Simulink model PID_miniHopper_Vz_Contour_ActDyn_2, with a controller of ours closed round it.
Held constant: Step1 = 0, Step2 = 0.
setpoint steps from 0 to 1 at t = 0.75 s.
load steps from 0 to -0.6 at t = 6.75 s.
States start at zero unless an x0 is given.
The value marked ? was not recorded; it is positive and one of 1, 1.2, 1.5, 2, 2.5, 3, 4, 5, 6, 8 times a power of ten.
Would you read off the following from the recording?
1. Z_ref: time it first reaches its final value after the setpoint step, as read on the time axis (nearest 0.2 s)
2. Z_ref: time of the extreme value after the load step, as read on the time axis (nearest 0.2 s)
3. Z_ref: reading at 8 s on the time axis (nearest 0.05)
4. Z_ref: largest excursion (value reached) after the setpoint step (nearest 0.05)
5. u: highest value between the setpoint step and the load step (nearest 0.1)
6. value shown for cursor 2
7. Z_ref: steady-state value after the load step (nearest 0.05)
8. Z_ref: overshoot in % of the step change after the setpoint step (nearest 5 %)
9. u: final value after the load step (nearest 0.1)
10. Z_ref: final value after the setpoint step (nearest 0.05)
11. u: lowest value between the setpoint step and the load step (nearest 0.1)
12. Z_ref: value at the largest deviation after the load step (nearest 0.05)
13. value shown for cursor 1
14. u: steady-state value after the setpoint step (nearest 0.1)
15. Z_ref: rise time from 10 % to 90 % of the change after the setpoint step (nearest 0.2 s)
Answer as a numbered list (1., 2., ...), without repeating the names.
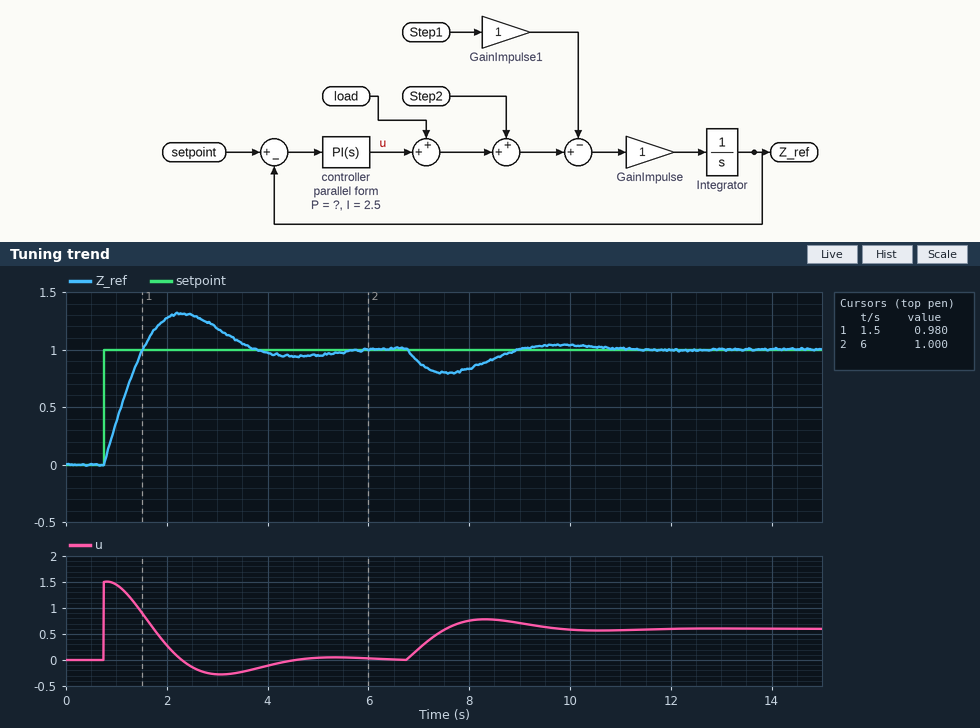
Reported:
1. 1.6 s
2. 7.6 s
3. 0.85
4. 1.30
5. 1.5
6. 1.000
7. 1.00
8. 30 %
9. 0.6
10. 1.00
11. -0.3
12. 0.80
13. 0.980
14. 0.0
15. 0.6 s
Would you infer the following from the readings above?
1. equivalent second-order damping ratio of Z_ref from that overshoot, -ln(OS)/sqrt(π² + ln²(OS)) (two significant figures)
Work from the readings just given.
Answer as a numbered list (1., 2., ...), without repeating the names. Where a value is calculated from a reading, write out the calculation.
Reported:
1. ln(0.3) = -1.204; 1.204 / sqrt(9.870 + 1.450) = 0.36
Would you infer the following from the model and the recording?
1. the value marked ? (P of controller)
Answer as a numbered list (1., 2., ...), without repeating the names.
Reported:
1. 1.5
